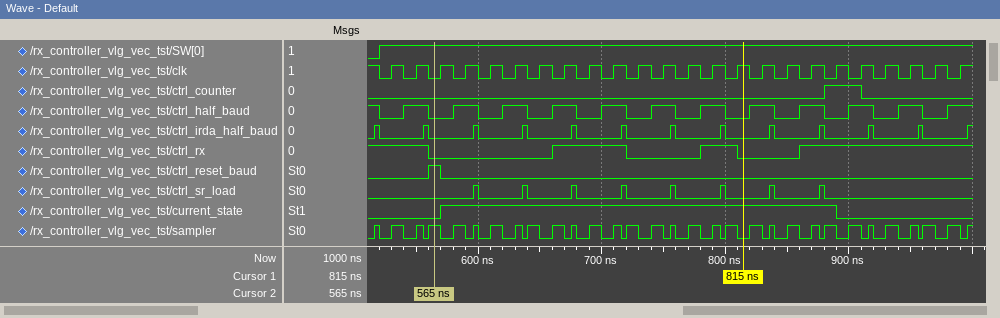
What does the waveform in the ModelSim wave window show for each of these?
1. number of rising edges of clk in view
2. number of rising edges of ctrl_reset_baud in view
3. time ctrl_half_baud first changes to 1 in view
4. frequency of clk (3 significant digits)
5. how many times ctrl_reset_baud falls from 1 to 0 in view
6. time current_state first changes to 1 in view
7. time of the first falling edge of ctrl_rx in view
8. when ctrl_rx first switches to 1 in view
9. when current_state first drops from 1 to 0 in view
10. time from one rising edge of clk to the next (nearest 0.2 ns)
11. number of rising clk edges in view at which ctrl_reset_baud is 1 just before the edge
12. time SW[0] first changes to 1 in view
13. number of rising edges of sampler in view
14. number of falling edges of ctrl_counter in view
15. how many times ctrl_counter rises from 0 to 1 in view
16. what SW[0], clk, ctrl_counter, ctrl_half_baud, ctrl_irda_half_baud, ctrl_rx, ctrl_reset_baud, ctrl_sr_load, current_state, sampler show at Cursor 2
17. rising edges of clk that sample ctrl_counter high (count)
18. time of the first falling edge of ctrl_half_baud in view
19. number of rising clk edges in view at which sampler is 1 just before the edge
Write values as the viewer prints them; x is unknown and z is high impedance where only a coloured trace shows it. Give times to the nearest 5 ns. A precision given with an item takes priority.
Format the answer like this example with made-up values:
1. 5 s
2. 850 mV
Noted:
1. 24
2. 1
3. 540 ns
4. 50.0 MHz
5. 1
6. 570 ns
7. 560 ns
8. 660 ns
9. 890 ns
10. 20 ns
11. 1
12. 520 ns
13. 31
14. 1
15. 1
16. SW[0]=1, clk=0, ctrl_counter=0, ctrl_half_baud=0, ctrl_irda_half_baud=0, ctrl_rx=0, ctrl_reset_baud=1, ctrl_sr_load=0, current_state=0, sampler=1
17. 2
18. 520 ns
19. 12
